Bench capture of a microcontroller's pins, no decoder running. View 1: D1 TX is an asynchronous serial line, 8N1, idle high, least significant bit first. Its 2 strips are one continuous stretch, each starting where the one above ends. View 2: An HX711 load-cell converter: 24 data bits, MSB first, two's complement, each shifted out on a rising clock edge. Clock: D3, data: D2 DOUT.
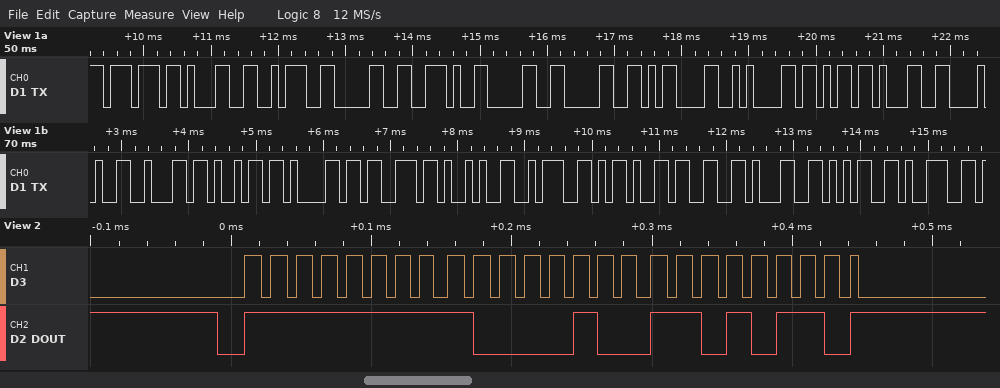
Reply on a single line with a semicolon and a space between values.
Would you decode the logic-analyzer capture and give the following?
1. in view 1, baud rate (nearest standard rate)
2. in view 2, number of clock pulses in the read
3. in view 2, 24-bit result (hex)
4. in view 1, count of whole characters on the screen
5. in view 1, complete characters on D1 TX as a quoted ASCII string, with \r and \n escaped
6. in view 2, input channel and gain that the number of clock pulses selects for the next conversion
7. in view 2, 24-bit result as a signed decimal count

9600 baud; 25; 0xFF84D6; 23; "w1:0.00\r\nk1(bias):-3159"; channel A, gain 128; -31530
